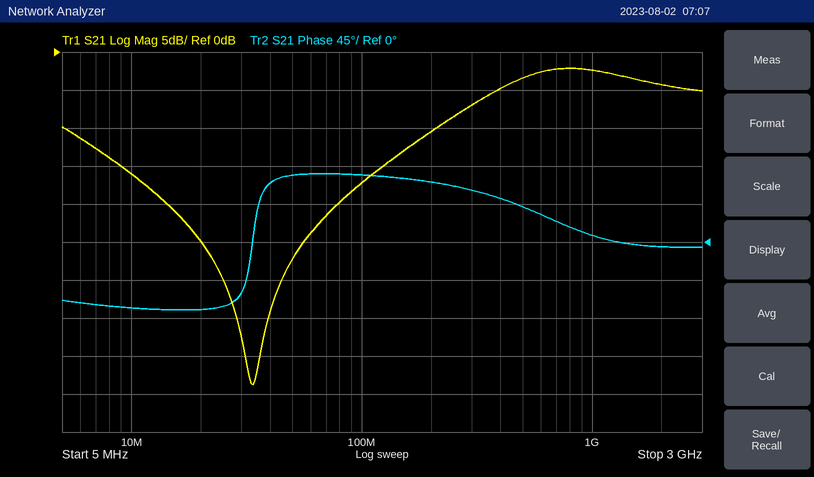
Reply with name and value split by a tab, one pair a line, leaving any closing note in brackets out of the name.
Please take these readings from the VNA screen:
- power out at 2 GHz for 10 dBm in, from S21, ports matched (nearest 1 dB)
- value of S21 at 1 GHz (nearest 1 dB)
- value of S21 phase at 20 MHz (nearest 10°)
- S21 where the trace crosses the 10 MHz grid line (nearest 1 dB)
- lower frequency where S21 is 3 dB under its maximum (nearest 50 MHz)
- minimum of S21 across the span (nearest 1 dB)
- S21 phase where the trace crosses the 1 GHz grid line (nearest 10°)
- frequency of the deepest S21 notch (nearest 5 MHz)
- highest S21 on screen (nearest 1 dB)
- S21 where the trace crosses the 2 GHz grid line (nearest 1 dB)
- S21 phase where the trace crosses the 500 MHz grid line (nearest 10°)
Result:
power out at 2 GHz for 10 dBm in, from S21, ports matched	6 dBm
value of S21 at 1 GHz	-2 dB
value of S21 phase at 20 MHz	-80°
S21 where the trace crosses the 10 MHz grid line	-16 dB
lower frequency where S21 is 3 dB under its maximum	400 MHz
minimum of S21 across the span	-44 dB
S21 phase where the trace crosses the 1 GHz grid line	10°
frequency of the deepest S21 notch	35 MHz
highest S21 on screen	-2 dB
S21 where the trace crosses the 2 GHz grid line	-4 dB
S21 phase where the trace crosses the 500 MHz grid line	40°
